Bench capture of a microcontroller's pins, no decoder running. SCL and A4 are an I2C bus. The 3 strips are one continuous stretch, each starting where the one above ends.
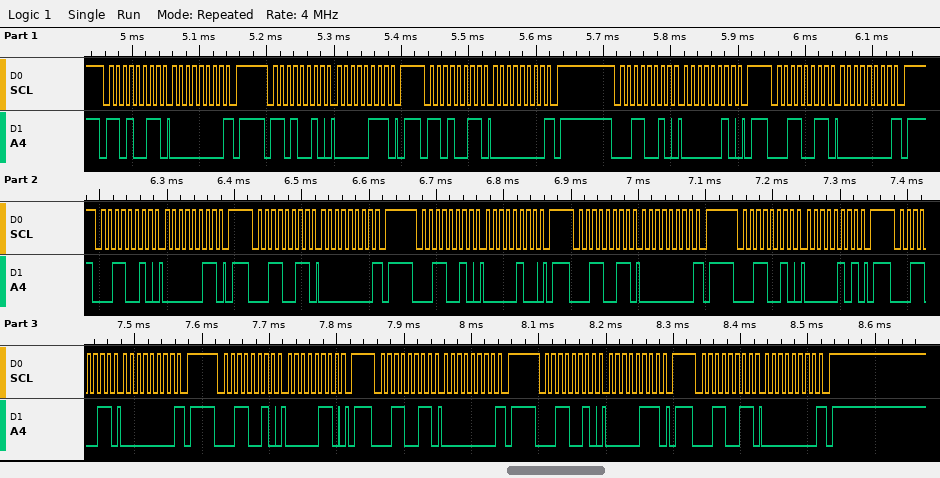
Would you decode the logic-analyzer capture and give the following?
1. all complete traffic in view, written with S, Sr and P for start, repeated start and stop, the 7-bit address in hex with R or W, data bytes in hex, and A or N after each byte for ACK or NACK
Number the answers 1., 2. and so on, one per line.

1. S 69R A 00 N P S 69W A 07 A P S 69R A 00 N P S 19W A 02 A P S 19R A 00 N P S 19W A 03 A P S 19R A 00 N P S 19W A 04 A P S 19R A 00 N P S 19W A 05 A P S 19R A 00 N P S 19W A 06 A P S 19R A 00 N P S 19W A 07 A P S 19R A 00 N P
